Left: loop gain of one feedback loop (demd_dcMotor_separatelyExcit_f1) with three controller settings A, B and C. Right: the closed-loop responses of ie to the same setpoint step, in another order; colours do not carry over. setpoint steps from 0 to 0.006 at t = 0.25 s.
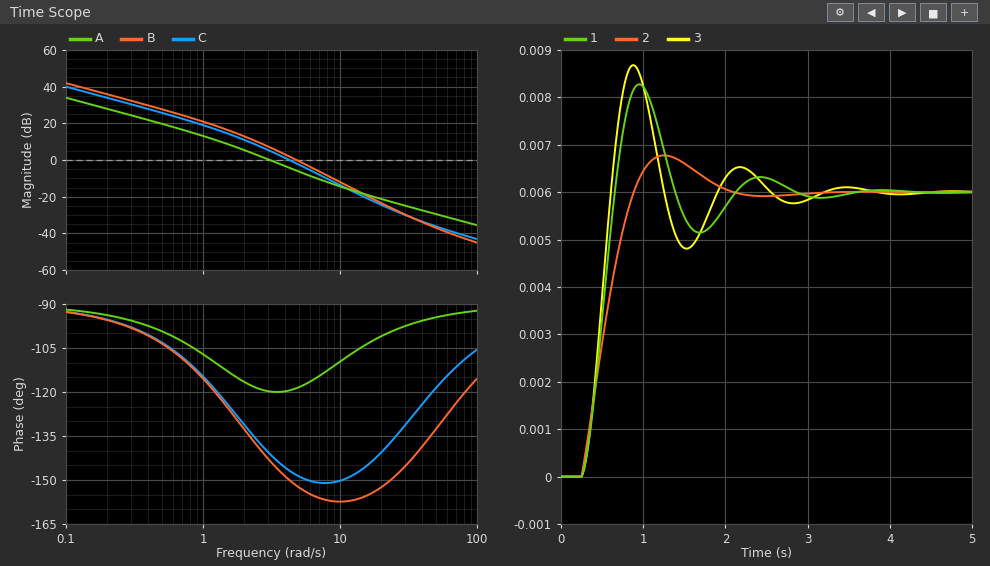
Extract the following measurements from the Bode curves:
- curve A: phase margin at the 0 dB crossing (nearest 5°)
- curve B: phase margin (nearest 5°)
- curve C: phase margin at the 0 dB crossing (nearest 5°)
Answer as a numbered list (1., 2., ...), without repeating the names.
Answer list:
1. 60°
2. 30°
3. 35°
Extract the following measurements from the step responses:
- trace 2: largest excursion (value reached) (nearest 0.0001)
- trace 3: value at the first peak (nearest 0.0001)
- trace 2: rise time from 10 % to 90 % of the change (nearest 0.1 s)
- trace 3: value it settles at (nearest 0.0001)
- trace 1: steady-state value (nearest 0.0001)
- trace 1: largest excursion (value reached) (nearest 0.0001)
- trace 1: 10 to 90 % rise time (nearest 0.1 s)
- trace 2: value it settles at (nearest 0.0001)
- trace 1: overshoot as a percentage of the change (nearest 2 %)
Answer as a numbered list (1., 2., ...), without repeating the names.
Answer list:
1. 0.0068
2. 0.0087
3. 0.5 s
4. 0.0060
5. 0.0060
6. 0.0083
7. 0.3 s
8. 0.0060
9. 38 %
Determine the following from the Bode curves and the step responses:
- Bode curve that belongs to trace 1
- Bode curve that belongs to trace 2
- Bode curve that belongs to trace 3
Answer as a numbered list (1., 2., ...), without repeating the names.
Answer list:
1. C
2. A
3. B
